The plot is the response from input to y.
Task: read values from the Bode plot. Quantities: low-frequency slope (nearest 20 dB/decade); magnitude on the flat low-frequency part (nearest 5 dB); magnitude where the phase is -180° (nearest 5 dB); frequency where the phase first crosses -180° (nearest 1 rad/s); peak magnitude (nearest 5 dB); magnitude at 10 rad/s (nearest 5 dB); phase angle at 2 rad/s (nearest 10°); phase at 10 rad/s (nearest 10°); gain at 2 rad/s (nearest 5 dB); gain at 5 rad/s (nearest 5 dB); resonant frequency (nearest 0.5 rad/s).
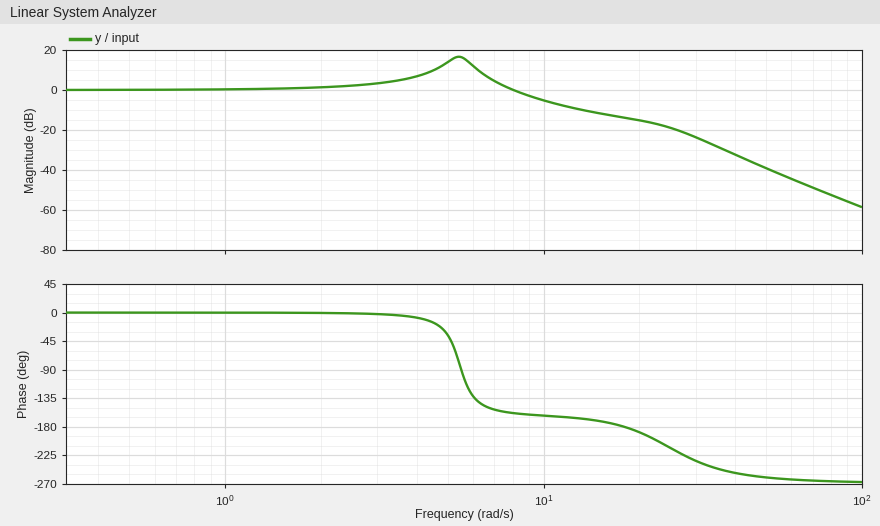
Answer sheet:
0 dB/decade
0 dB
-15 dB
18 rad/s
15 dB
-5 dB
0°
-160°
0 dB
15 dB
5.5 rad/s
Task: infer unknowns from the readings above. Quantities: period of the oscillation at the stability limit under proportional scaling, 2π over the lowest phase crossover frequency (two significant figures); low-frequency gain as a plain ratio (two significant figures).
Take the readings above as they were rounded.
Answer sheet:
0.35 s
1.0
